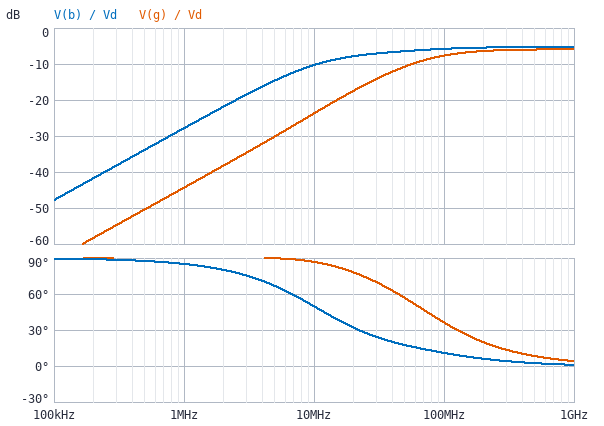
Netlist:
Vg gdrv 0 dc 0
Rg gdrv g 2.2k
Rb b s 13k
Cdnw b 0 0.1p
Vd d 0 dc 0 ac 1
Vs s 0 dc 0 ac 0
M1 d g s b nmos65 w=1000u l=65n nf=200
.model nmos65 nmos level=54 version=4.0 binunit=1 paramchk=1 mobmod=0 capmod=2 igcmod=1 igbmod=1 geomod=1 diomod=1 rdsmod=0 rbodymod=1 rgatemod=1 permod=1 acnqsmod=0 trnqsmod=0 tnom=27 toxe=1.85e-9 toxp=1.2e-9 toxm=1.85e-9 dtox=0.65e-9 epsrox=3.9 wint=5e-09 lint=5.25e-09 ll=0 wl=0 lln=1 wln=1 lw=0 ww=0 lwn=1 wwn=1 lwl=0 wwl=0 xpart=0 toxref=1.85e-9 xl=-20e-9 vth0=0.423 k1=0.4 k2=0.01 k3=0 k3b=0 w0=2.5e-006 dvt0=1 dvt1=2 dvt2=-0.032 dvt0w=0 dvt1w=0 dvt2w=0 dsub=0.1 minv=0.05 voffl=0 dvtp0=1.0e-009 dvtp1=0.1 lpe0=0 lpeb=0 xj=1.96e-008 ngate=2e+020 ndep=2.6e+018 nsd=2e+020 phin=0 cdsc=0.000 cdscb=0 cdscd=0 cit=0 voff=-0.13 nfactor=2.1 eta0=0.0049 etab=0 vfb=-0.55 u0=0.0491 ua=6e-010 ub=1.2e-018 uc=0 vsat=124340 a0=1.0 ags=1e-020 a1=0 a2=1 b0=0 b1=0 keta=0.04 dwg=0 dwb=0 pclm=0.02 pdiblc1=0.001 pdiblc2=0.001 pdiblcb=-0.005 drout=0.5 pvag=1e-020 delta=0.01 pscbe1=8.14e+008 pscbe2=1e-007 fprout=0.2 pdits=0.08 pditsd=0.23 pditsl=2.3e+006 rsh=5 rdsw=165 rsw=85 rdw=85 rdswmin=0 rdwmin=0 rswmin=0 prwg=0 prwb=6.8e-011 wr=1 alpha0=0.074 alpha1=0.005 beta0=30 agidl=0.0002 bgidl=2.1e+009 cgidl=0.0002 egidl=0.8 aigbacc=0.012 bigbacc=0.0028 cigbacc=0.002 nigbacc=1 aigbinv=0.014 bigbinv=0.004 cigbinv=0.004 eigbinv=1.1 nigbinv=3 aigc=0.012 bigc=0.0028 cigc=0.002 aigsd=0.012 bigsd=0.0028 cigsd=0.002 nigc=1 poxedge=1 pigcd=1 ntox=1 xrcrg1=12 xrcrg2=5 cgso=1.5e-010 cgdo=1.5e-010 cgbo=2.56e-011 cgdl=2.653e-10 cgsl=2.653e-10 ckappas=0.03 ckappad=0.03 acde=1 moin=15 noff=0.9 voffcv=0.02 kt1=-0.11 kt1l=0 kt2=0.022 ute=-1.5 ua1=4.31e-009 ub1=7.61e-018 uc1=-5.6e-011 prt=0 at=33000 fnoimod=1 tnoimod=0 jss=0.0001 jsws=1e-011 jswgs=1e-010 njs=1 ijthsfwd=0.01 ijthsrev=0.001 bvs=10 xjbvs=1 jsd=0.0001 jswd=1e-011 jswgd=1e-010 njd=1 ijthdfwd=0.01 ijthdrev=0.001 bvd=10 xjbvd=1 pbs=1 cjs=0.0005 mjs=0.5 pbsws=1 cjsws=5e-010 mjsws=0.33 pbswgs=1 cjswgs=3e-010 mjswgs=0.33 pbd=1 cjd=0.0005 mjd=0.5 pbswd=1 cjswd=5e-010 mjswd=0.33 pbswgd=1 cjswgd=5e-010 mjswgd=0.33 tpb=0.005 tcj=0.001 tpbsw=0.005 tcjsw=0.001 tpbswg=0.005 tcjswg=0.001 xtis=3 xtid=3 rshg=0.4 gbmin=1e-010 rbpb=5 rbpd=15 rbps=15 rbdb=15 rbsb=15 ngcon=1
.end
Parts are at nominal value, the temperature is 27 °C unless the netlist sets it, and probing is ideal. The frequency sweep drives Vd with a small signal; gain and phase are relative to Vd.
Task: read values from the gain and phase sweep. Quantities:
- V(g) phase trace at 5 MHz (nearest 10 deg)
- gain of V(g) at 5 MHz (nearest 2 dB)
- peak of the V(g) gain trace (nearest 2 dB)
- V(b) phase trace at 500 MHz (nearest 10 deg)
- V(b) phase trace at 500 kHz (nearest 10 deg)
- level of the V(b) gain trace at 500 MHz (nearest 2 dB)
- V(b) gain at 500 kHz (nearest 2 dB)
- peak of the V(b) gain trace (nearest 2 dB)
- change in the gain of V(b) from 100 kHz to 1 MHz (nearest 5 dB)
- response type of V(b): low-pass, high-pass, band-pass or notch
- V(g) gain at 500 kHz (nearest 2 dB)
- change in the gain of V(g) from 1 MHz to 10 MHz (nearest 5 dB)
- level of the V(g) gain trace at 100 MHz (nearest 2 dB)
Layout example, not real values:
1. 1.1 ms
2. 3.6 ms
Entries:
1. 90 deg
2. -30 dB
3. -6 dB
4. 0 deg
5. 90 deg
6. -6 dB
7. -34 dB
8. -6 dB
9. 20 dB
10. high-pass
11. -50 dB
12. 20 dB
13. -8 dB
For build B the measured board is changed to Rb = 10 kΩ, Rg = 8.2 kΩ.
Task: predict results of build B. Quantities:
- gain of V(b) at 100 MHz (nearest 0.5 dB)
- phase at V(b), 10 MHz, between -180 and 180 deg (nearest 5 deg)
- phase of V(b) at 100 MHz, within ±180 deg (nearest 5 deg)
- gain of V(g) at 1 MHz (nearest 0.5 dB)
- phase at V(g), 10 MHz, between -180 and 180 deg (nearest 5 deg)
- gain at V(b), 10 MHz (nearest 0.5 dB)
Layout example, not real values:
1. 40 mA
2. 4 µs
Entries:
1. -5.5 dB
2. 60 deg
3. 10 deg
4. -33.0 dB
5. 65 deg
6. -11.5 dB
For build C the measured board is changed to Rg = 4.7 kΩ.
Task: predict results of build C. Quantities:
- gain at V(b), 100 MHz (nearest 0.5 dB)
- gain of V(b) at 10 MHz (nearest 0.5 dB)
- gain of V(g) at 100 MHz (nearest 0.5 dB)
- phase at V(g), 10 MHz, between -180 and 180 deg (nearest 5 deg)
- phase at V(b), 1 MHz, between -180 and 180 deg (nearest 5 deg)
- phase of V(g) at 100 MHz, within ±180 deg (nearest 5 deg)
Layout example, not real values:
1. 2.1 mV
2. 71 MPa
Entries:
1. -5.5 dB
2. -10.0 dB
3. -6.5 dB
4. 80 deg
5. 85 deg
6. 20 deg
